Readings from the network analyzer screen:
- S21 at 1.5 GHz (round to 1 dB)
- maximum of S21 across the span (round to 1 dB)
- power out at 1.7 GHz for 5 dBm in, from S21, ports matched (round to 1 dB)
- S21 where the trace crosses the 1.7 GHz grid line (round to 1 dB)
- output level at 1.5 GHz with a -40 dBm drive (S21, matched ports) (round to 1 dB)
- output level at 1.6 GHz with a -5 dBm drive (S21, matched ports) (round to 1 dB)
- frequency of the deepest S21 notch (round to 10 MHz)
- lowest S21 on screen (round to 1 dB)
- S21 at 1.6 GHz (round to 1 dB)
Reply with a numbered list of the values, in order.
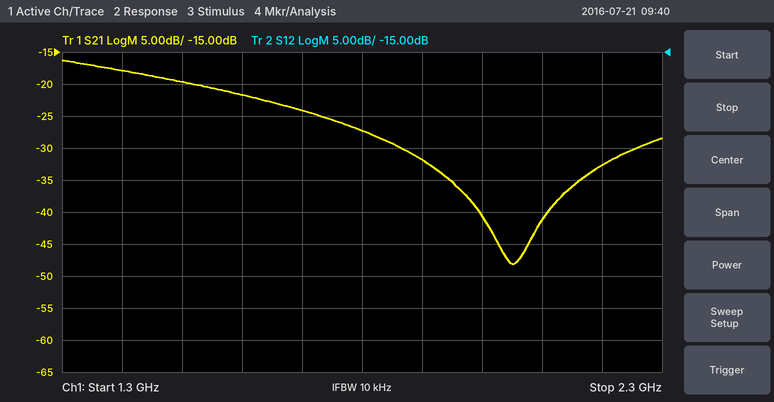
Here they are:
1. -20 dB
2. -16 dB
3. -19 dBm
4. -24 dB
5. -60 dBm
6. -27 dBm
7. 2.05 GHz
8. -48 dB
9. -22 dB
